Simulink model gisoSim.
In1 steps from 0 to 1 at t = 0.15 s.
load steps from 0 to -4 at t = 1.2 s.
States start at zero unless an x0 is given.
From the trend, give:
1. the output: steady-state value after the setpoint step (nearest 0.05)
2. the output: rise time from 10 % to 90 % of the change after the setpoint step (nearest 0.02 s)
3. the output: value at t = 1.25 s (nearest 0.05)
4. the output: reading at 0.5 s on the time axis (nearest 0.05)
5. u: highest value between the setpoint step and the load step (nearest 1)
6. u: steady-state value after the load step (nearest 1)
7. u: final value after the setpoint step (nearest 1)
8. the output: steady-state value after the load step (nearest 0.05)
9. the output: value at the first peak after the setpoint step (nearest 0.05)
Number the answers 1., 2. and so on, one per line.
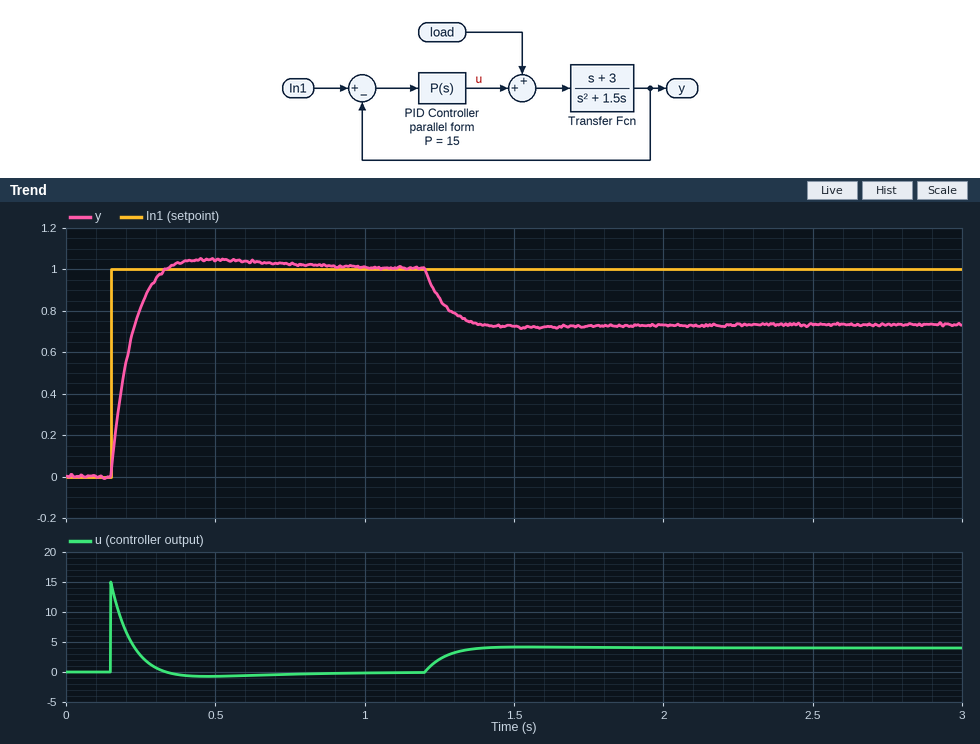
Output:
1. 1.00
2. 0.12 s
3. 0.85
4. 1.05
5. 15
6. 4
7. 0
8. 0.75
9. 1.05
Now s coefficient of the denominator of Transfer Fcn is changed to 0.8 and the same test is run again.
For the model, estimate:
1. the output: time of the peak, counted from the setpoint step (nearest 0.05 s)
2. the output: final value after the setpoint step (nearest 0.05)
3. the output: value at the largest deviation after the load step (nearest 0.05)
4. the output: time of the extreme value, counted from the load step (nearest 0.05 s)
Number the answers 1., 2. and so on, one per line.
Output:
1. 0.30 s
2. 1.00
3. 0.70
4. 0.30 s
